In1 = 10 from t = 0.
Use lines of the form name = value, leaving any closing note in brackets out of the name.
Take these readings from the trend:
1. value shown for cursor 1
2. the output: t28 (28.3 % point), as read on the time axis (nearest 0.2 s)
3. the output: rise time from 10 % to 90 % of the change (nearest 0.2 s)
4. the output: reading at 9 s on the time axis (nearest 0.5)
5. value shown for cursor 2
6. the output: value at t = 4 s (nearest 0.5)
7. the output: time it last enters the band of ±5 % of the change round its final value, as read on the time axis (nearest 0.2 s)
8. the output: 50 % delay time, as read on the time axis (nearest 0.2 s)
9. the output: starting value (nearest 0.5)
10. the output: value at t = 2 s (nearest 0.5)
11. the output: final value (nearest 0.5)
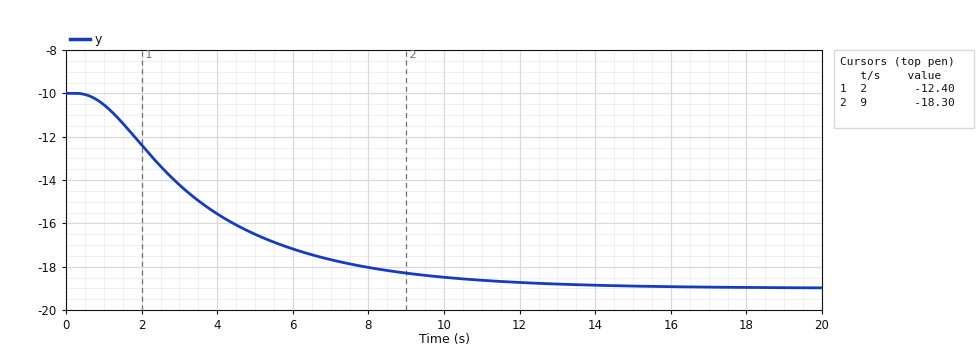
value shown for cursor 1 = -12.40
the output: t28 (28.3 % point), as read on the time axis = 2.0 s
the output: rise time from 10 % to 90 % of the change = 7.0 s
the output: reading at 9 s on the time axis = -18.5
value shown for cursor 2 = -18.30
the output: value at t = 4 s = -15.5
the output: time it last enters the band of ±5 % of the change round its final value, as read on the time axis = 10.4 s
the output: 50 % delay time, as read on the time axis = 3.2 s
the output: starting value = -10.0
the output: value at t = 2 s = -12.5
the output: final value = -19.0
